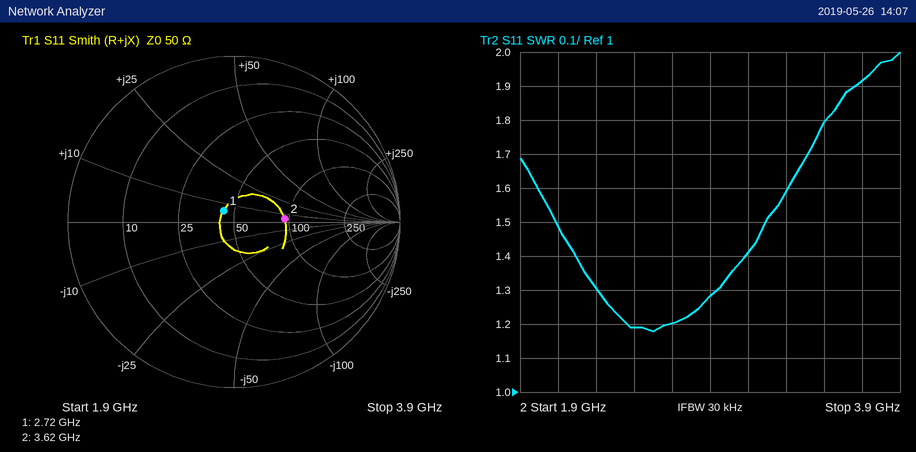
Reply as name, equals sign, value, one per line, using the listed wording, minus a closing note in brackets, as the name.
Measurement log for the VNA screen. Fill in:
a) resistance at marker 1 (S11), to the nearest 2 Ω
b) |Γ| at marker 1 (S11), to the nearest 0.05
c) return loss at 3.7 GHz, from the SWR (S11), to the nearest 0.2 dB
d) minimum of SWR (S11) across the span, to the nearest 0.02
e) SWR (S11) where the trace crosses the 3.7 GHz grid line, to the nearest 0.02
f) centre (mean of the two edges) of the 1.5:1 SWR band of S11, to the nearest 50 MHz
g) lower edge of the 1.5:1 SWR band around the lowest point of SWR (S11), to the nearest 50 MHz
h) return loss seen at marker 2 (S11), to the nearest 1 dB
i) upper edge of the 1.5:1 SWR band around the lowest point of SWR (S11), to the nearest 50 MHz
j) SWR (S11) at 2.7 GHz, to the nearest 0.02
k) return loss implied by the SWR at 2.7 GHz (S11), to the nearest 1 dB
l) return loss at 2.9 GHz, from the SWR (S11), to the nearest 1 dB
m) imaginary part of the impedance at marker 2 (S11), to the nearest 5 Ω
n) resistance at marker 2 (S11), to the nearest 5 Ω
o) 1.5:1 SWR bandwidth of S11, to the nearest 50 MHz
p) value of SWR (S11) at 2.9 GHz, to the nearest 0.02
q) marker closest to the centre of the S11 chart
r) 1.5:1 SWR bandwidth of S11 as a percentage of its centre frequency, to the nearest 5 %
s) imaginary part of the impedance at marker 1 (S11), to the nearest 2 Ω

resistance at marker 1 (S11), to the nearest 2 Ω = 44 Ω
|Γ| at marker 1 (S11), to the nearest 0.05 = 0.10
return loss at 3.7 GHz, from the SWR (S11), to the nearest 0.2 dB = 10.0 dB
minimum of SWR (S11) across the span, to the nearest 0.02 = 1.18
SWR (S11) where the trace crosses the 3.7 GHz grid line, to the nearest 0.02 = 1.92
centre (mean of the two edges) of the 1.5:1 SWR band of S11, to the nearest 50 MHz = 2.65 GHz
lower edge of the 1.5:1 SWR band around the lowest point of SWR (S11), to the nearest 50 MHz = 2.10 GHz
return loss seen at marker 2 (S11), to the nearest 1 dB = 10 dB
upper edge of the 1.5:1 SWR band around the lowest point of SWR (S11), to the nearest 50 MHz = 3.20 GHz
SWR (S11) at 2.7 GHz, to the nearest 0.02 = 1.20
return loss implied by the SWR at 2.7 GHz (S11), to the nearest 1 dB = 21 dB
return loss at 2.9 GHz, from the SWR (S11), to the nearest 1 dB = 18 dB
imaginary part of the impedance at marker 2 (S11), to the nearest 5 Ω = +5 Ω
resistance at marker 2 (S11), to the nearest 5 Ω = 95 Ω
1.5:1 SWR bandwidth of S11, to the nearest 50 MHz = 1.10 GHz
value of SWR (S11) at 2.9 GHz, to the nearest 0.02 = 1.28
marker closest to the centre of the S11 chart = marker 1
1.5:1 SWR bandwidth of S11 as a percentage of its centre frequency, to the nearest 5 % = 40 %
imaginary part of the impedance at marker 1 (S11), to the nearest 2 Ω = +6 Ω
